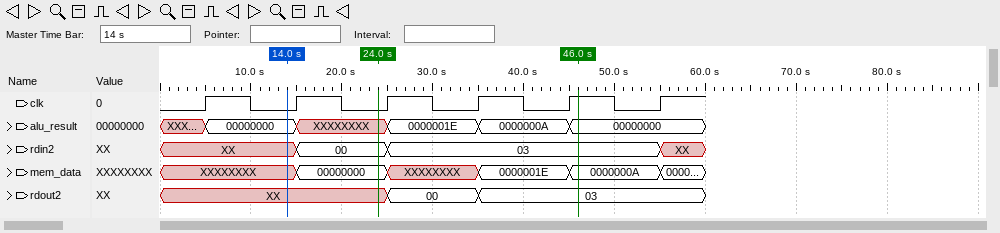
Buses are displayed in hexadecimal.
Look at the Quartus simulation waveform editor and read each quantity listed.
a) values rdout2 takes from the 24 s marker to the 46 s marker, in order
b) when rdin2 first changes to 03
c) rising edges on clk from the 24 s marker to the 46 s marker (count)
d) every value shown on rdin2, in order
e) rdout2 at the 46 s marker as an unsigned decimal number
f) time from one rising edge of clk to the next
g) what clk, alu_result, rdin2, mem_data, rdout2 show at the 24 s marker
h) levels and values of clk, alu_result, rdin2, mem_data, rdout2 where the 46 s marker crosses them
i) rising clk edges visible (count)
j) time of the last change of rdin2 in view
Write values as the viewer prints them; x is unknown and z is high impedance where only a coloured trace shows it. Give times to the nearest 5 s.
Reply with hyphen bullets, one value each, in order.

- XX, 00, 03
- 25 s
- 3
- XX, 00, 03, XX
- 3
- 10 s
- clk=0, alu_result=XXXXXXXX, rdin2=00, mem_data=00000000, rdout2=XX
- clk=1, alu_result=00000000, rdin2=03, mem_data=0000000A, rdout2=03
- 6
- 55 s
